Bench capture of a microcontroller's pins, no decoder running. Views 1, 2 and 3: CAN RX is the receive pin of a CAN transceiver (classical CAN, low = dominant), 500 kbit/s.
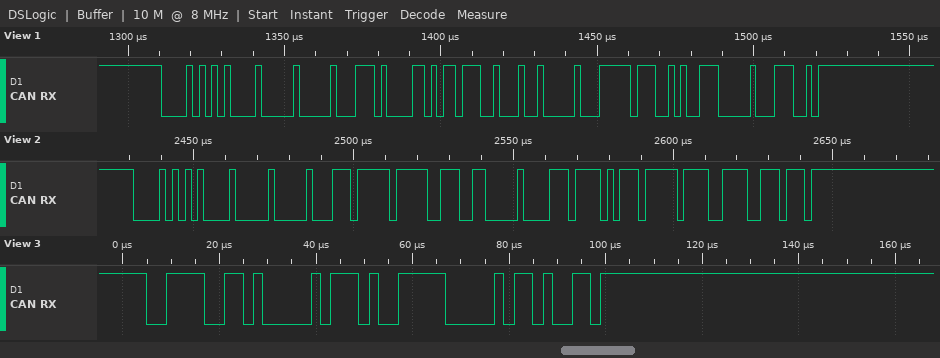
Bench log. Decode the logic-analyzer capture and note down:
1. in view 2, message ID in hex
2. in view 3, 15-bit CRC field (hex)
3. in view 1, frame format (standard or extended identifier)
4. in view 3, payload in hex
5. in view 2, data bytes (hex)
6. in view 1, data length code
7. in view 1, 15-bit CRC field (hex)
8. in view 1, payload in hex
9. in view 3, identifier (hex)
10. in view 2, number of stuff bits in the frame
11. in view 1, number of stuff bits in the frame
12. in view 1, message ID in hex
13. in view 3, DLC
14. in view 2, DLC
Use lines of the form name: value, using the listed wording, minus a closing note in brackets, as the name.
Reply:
in view 2, message ID in hex: 0x0AA
in view 3, 15-bit CRC field: 0x7069
in view 1, frame format: standard
in view 3, payload in hex: D3
in view 2, data bytes: 00 3B FF 73 00 77 AE FF
in view 1, data length code: 8
in view 1, 15-bit CRC field: 0x601C
in view 1, payload in hex: 00 3A 1A DC 89 00 FF 29
in view 3, identifier: 0x3CD
in view 2, number of stuff bits in the frame: 6
in view 1, number of stuff bits in the frame: 5
in view 1, message ID in hex: 0x0AA
in view 3, DLC: 1
in view 2, DLC: 8
